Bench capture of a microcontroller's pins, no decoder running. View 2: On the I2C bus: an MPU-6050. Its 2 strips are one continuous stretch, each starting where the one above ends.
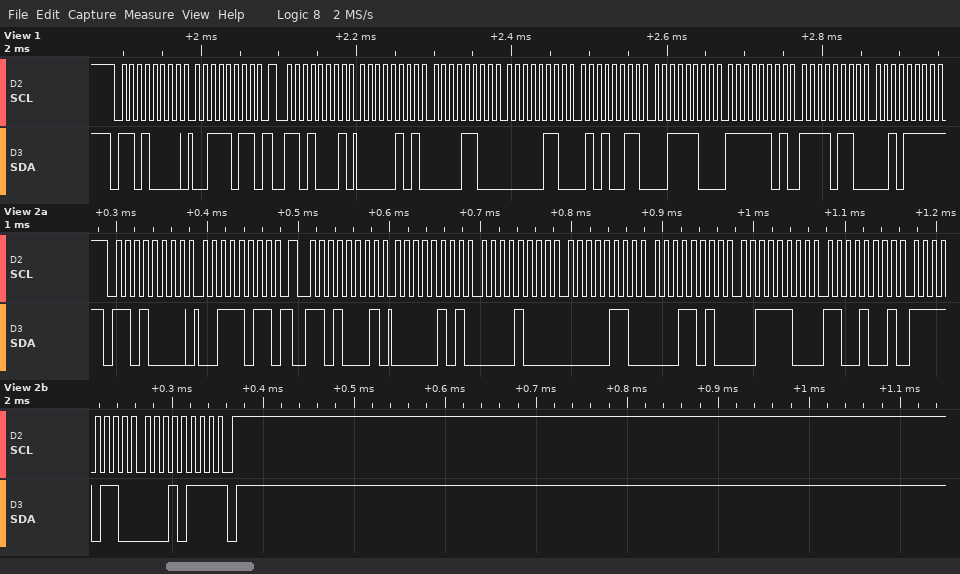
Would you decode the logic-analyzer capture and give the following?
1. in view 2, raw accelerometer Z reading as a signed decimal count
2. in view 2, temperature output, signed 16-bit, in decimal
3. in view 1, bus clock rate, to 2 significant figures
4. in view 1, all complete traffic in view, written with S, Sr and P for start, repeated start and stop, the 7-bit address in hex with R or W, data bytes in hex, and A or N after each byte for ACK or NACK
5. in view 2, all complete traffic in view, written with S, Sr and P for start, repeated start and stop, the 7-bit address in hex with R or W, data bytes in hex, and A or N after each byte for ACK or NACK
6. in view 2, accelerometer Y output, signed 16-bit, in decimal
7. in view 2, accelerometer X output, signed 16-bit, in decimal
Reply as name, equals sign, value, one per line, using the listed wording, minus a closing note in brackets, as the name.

in view 2, raw accelerometer Z reading as a signed decimal count = 15561
in view 2, temperature output, signed 16-bit, in decimal = -2537
in view 1, bus clock rate, to 2 significant figures = 100 kHz
in view 1, all complete traffic in view, written with S, Sr and P for start, repeated start and stop, the 7-bit address in hex with R or W, data bytes in hex, and A or N after each byte for ACK or NACK = S 68W A 3B A Sr 68R A 05 A 0C A 06 A 53 A 3C A FD A F6 A 2F N
in view 2, all complete traffic in view, written with S, Sr and P for start, repeated start and stop, the 7-bit address in hex with R or W, data bytes in hex, and A or N after each byte for ACK or NACK = S 68W A 3B A Sr 68R A 05 A 08 A 06 A 1A A 3C A C9 A F6 A 17 N P
in view 2, accelerometer Y output, signed 16-bit, in decimal = 1562
in view 2, accelerometer X output, signed 16-bit, in decimal = 1288
